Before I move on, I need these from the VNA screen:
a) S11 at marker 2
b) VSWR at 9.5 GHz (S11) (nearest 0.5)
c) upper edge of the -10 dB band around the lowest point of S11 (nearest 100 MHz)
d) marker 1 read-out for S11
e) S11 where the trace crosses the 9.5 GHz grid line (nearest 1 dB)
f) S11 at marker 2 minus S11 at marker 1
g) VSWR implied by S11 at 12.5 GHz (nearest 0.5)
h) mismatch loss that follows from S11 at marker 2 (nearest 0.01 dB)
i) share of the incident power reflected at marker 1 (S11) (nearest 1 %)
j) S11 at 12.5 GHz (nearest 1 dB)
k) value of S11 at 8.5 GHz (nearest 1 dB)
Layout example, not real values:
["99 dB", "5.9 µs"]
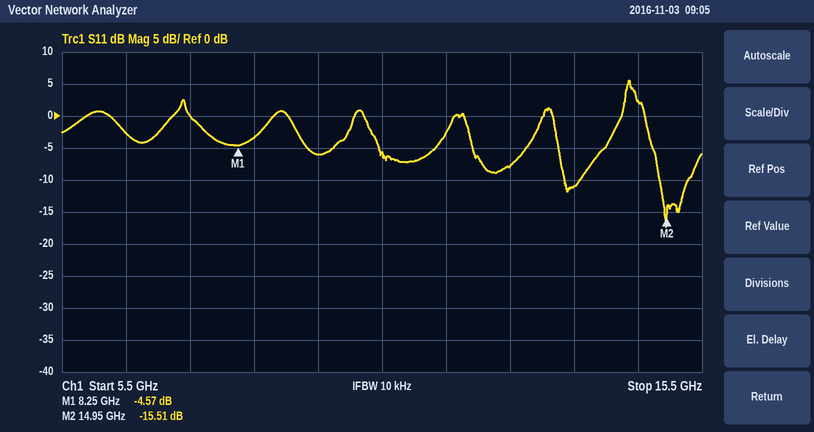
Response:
["-15.51 dB", "3.0", "15.3 GHz", "-4.57 dB", "-6 dB", "-10.94 dB", "2.5", "0.12 dB", "35 %", "-8 dB", "-3 dB"]
